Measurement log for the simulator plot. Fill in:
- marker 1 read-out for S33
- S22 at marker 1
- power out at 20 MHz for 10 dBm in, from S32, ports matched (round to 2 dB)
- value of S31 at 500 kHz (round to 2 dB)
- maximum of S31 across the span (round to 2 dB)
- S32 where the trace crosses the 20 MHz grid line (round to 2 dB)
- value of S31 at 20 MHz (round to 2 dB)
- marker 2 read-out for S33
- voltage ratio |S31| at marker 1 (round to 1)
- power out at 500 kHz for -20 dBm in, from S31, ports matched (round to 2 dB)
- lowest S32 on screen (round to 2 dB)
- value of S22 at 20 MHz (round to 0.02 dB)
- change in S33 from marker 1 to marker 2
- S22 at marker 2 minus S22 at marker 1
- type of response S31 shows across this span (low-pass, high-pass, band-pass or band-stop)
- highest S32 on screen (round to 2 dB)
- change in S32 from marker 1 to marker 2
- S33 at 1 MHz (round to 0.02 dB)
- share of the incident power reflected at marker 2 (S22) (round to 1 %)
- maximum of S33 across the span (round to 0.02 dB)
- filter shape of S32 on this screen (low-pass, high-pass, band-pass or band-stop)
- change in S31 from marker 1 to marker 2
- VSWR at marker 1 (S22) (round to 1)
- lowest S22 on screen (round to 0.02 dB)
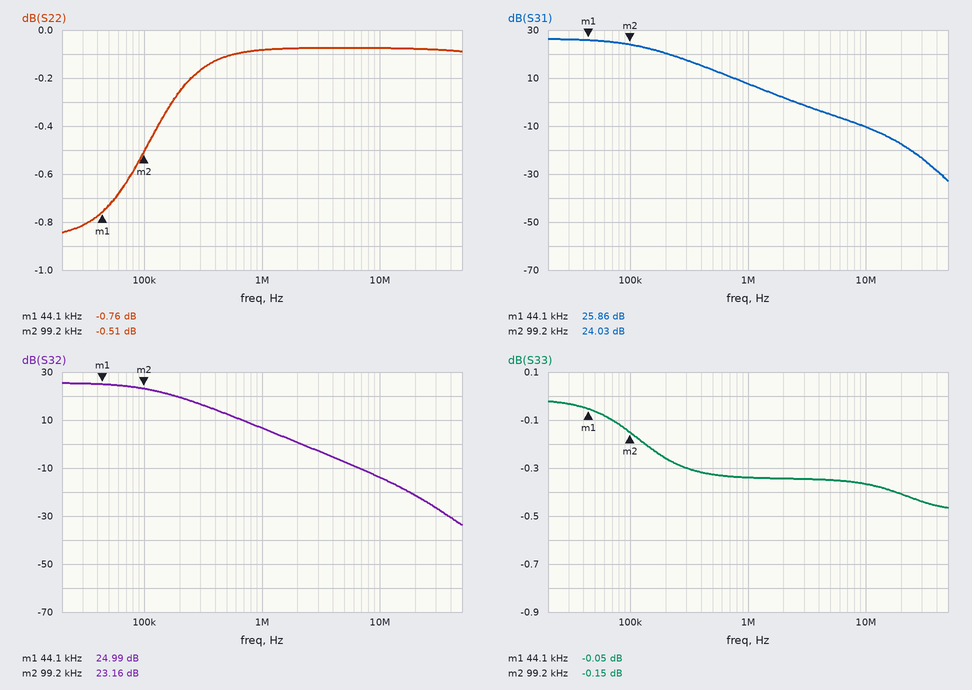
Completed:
-0.05 dB
-0.76 dB
-12 dBm
14 dB
26 dB
-22 dB
-18 dB
-0.15 dB
20
-6 dBm
-34 dB
-0.08 dB
-0.10 dB
0.25 dB
low-pass
26 dB
-1.83 dB
-0.34 dB
89 %
-0.02 dB
low-pass
-1.83 dB
23
-0.84 dB
